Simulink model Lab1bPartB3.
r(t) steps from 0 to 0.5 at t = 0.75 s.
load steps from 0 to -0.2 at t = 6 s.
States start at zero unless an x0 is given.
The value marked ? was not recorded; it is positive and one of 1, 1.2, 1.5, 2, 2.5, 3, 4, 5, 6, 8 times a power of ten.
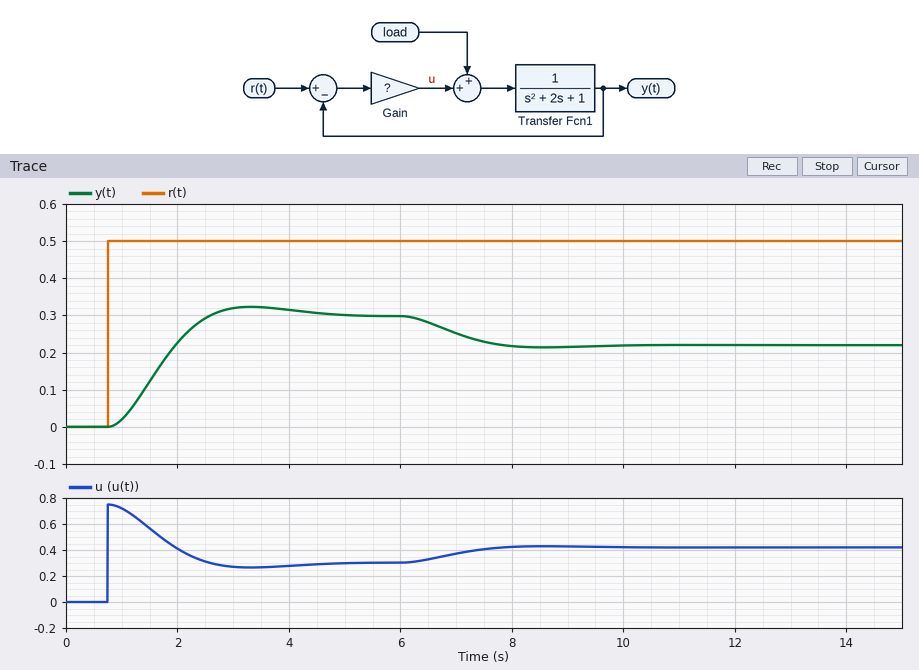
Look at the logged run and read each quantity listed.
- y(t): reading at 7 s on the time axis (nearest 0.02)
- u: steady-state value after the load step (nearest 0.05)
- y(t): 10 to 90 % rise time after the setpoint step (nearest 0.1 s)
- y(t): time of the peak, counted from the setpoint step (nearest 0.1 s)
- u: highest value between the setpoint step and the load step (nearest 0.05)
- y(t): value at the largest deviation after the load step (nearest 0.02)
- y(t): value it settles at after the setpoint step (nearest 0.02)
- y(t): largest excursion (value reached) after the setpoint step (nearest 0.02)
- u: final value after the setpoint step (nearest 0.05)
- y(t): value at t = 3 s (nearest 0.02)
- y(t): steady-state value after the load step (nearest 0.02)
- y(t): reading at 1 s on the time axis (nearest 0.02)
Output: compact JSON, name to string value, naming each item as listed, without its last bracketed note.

{"y(t): reading at 7 s on the time axis": "0.26", "u: steady-state value after the load step": "0.40", "y(t): 10 to 90 % rise time after the setpoint step": "1.2 s", "y(t): time of the peak, counted from the setpoint step": "2.6 s", "u: highest value between the setpoint step and the load step": "0.75", "y(t): value at the largest deviation after the load step": "0.22", "y(t): value it settles at after the setpoint step": "0.30", "y(t): largest excursion (value reached) after the setpoint step": "0.32", "u: final value after the setpoint step": "0.30", "y(t): value at t = 3 s": "0.32", "y(t): steady-state value after the load step": "0.22", "y(t): reading at 1 s on the time axis": "0.02"}
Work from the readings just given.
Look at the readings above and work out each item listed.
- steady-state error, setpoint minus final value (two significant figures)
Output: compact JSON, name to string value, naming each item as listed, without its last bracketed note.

{"steady-state error, setpoint minus final value": "0.20"}
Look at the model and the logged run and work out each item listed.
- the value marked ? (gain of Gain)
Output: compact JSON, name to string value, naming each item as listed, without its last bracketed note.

{"the value marked ?": "1.5"}
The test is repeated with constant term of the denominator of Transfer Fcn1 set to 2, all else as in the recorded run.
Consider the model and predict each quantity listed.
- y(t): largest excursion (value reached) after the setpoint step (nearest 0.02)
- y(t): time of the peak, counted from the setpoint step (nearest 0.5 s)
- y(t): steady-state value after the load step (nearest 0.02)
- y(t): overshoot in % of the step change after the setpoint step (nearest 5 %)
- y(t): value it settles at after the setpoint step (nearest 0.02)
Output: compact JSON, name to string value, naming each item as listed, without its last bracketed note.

{"y(t): largest excursion (value reached) after the setpoint step": "0.24", "y(t): time of the peak, counted from the setpoint step": "2.0 s", "y(t): steady-state value after the load step": "0.16", "y(t): overshoot in % of the step change after the setpoint step": "15 %", "y(t): value it settles at after the setpoint step": "0.22"}
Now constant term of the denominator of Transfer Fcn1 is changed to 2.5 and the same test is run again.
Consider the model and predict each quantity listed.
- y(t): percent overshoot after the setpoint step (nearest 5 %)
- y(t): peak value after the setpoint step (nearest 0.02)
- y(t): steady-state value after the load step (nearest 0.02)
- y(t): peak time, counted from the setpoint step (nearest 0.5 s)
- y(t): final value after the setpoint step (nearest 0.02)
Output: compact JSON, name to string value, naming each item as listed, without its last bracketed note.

{"y(t): percent overshoot after the setpoint step": "15 %", "y(t): peak value after the setpoint step": "0.22", "y(t): steady-state value after the load step": "0.14", "y(t): peak time, counted from the setpoint step": "2.0 s", "y(t): final value after the setpoint step": "0.18"}
